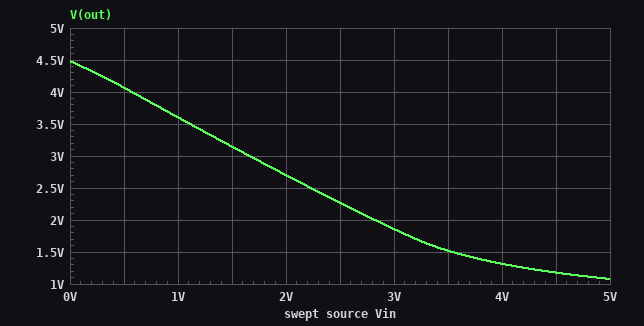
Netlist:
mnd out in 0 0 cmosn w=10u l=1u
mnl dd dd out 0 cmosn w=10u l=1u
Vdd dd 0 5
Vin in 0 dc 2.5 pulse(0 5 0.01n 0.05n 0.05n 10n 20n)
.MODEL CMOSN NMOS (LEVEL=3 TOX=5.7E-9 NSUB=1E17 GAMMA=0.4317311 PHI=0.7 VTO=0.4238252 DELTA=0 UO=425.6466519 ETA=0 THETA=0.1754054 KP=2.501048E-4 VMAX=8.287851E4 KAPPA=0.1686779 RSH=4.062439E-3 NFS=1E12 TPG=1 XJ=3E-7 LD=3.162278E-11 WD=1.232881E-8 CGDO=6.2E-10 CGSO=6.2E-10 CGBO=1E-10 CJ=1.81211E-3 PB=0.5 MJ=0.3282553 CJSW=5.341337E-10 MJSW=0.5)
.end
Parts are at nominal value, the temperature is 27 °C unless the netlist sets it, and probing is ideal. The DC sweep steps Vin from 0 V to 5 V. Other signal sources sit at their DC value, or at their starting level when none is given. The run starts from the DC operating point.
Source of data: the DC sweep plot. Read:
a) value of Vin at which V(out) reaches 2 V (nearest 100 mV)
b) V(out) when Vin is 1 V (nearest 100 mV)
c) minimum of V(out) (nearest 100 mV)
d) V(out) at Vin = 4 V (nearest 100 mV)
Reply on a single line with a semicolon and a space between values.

2.8 V; 3.6 V; 1.1 V; 1.3 V
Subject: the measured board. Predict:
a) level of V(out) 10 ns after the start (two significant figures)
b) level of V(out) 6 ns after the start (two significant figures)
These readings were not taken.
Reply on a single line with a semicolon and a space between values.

1.1 V; 1.1 V
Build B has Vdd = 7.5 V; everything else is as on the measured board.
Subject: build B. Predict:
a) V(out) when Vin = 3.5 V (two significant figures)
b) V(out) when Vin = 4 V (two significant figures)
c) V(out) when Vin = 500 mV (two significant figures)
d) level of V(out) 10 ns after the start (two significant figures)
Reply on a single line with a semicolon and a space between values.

3.7 V; 3.3 V; 6.4 V; 2.5 V
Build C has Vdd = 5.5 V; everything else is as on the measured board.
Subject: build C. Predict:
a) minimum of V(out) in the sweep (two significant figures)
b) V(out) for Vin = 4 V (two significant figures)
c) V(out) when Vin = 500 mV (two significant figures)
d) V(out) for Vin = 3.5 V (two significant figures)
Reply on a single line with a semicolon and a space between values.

1.3 V; 1.6 V; 4.5 V; 1.9 V
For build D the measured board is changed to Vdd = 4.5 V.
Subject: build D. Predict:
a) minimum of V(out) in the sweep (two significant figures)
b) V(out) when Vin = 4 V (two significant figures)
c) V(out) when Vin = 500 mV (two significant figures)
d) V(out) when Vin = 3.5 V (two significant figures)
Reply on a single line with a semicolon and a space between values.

890 mV; 1.1 V; 3.6 V; 1.2 V
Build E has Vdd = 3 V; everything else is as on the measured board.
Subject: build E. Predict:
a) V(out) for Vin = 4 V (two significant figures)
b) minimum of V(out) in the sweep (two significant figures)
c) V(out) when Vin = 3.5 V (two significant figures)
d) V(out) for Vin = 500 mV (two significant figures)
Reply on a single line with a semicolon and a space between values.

500 mV; 430 mV; 550 mV; 2.2 V
